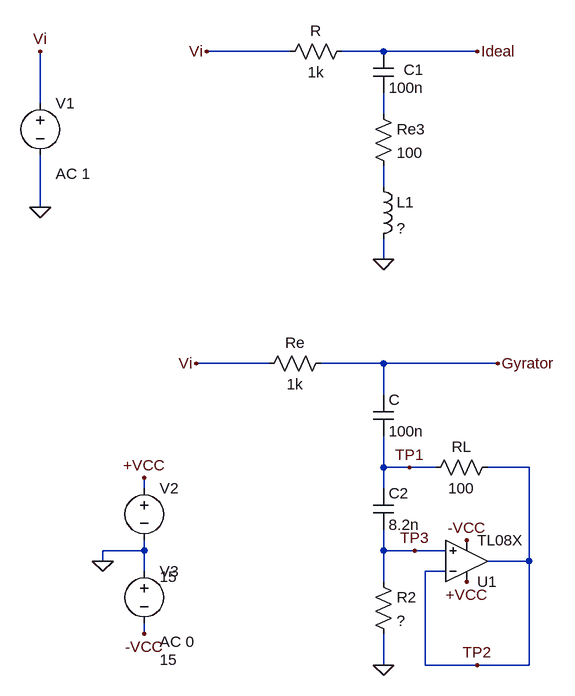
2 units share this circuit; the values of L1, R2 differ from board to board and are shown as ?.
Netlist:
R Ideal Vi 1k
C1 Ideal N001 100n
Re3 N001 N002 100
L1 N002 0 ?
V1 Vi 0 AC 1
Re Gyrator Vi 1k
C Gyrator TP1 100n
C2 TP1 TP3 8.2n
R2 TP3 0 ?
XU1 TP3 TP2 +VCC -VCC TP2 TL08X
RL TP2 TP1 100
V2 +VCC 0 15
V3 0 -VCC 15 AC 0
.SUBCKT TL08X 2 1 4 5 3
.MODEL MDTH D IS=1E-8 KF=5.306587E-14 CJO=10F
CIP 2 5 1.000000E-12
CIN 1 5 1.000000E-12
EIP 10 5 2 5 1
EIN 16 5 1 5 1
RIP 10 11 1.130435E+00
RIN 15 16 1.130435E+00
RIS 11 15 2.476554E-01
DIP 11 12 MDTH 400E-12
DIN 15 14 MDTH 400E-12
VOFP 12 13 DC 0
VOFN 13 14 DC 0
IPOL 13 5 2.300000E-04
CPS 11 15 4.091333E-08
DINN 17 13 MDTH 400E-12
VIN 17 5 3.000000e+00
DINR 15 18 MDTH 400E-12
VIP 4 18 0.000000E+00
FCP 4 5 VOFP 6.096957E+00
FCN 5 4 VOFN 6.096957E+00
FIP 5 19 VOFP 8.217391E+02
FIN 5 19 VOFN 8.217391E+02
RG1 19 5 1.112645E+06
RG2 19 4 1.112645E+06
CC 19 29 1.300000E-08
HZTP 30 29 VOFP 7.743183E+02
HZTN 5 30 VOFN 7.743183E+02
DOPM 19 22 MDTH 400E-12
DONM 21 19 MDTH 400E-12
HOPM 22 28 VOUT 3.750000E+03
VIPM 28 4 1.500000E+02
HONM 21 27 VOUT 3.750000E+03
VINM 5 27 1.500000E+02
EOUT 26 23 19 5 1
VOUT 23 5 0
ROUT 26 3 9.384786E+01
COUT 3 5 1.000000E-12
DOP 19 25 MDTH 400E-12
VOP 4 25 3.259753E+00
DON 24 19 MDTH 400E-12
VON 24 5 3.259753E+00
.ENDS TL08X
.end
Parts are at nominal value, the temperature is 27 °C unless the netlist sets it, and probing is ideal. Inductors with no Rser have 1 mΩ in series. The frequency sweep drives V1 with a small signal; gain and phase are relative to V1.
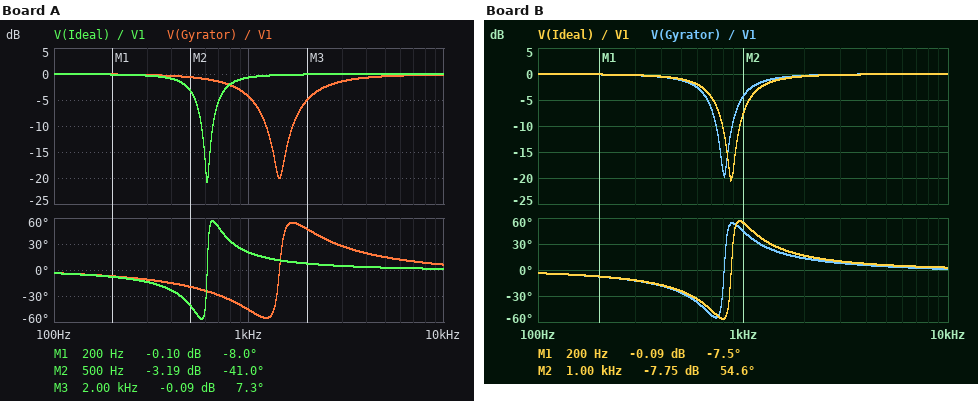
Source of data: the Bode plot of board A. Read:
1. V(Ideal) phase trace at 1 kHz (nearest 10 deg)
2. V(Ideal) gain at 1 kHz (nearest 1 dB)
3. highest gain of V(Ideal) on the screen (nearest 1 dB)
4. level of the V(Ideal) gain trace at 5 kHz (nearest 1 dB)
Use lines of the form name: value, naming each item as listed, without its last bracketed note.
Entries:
V(Ideal) phase trace at 1 kHz: 20 deg
V(Ideal) gain at 1 kHz: -1 dB
highest gain of V(Ideal) on the screen: 0 dB
level of the V(Ideal) gain trace at 5 kHz: 0 dB
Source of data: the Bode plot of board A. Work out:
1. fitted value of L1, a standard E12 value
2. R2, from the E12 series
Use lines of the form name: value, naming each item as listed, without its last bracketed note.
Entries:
fitted value of L1, a standard E12 value: 680 mH
R2, from the E12 series: 150 kΩ
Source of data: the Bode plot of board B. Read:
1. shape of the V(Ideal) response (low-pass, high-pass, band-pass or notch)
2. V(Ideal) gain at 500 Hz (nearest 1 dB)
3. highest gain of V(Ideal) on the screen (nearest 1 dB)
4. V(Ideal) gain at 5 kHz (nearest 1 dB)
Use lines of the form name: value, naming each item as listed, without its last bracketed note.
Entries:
shape of the V(Ideal) response: notch
V(Ideal) gain at 500 Hz: -1 dB
highest gain of V(Ideal) on the screen: 0 dB
V(Ideal) gain at 5 kHz: 0 dB
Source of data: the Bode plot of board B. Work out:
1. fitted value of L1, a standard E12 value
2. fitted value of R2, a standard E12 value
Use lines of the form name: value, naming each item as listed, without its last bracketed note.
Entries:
fitted value of L1, a standard E12 value: 330 mH
fitted value of R2, a standard E12 value: 470 kΩ
